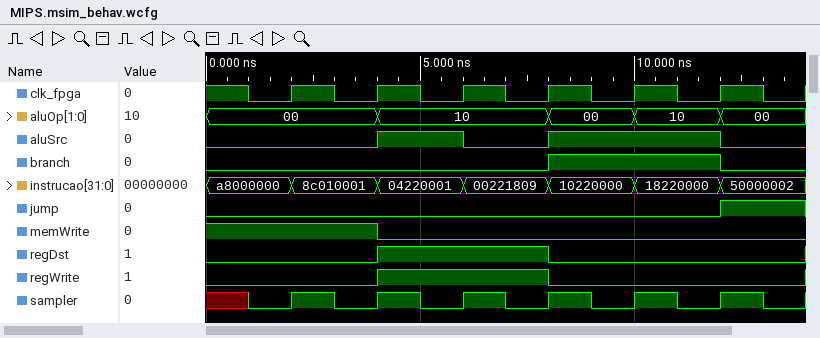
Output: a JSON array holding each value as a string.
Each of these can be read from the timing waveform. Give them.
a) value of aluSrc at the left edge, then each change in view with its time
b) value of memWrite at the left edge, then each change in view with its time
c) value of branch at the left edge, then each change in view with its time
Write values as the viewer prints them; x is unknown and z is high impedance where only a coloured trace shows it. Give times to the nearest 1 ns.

["0, 1 at 4 ns, 0 at 6 ns, 1 at 8 ns, 0 at 12 ns", "1, 0 at 4 ns", "0, 1 at 8 ns, 0 at 12 ns"]
